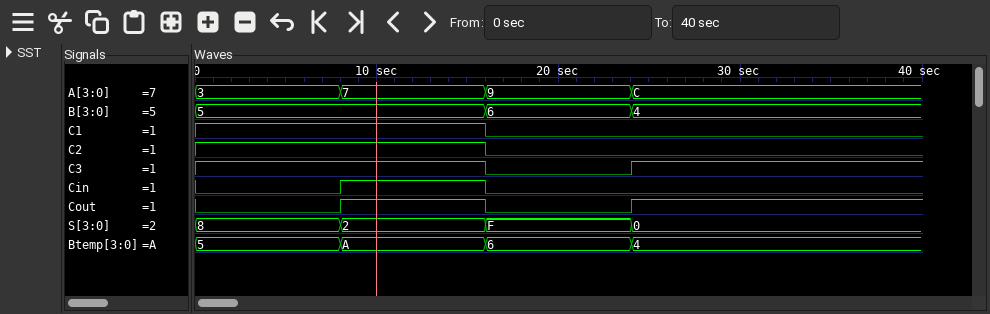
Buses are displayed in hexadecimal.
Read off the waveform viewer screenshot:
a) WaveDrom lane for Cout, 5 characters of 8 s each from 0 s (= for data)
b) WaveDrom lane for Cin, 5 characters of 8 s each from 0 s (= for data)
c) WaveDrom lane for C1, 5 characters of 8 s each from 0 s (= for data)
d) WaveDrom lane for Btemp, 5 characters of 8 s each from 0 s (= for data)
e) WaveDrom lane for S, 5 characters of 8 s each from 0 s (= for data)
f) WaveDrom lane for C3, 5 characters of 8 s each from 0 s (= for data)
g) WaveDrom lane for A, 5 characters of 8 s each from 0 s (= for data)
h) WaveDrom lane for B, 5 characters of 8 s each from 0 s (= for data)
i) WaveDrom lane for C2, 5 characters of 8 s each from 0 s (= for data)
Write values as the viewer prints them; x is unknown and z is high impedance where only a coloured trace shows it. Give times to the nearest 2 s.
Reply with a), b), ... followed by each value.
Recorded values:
a) {name: 'Cout', wave: '0101.'}
b) {name: 'Cin', wave: '010..'}
c) {name: 'C1', wave: '1.0..'}
d) {name: 'Btemp', wave: '====.', data: '5 A 6 4'}
e) {name: 'S', wave: '====.', data: '8 2 F 0'}
f) {name: 'C3', wave: '1.01.'}
g) {name: 'A', wave: '====.', data: '3 7 9 C'}
h) {name: 'B', wave: '=.==.', data: '5 6 4'}
i) {name: 'C2', wave: '1.0..'}
